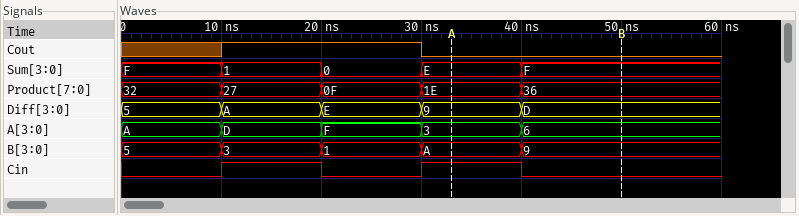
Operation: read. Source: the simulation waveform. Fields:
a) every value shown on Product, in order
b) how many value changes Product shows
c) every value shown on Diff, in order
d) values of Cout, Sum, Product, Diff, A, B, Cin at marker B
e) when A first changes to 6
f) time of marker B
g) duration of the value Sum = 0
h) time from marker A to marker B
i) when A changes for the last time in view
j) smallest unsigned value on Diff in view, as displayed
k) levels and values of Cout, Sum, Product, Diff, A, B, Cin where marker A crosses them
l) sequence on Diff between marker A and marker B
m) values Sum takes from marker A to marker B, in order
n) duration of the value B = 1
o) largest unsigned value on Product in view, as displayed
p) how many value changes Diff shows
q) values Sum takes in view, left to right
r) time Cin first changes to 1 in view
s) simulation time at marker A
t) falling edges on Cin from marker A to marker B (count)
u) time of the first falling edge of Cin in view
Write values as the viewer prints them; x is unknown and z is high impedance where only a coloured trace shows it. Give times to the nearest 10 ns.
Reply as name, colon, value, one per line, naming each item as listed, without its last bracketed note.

every value shown on Product, in order: 32, 27, 0F, 1E, 36
how many value changes Product shows: 4
every value shown on Diff, in order: 5, A, E, 9, D
values of Cout, Sum, Product, Diff, A, B, Cin at marker B: Cout=0, Sum=F, Product=36, Diff=D, A=6, B=9, Cin=0
when A first changes to 6: 40 ns
time of marker B: 50 ns
duration of the value Sum = 0: 10 ns
time from marker A to marker B: 20 ns
when A changes for the last time in view: 40 ns
smallest unsigned value on Diff in view, as displayed: 5
levels and values of Cout, Sum, Product, Diff, A, B, Cin where marker A crosses them: Cout=0, Sum=E, Product=1E, Diff=9, A=3, B=A, Cin=1
sequence on Diff between marker A and marker B: 9, D
values Sum takes from marker A to marker B, in order: E, F
duration of the value B = 1: 10 ns
largest unsigned value on Product in view, as displayed: 36
how many value changes Diff shows: 4
values Sum takes in view, left to right: F, 1, 0, E, F
time Cin first changes to 1 in view: 10 ns
simulation time at marker A: 30 ns
falling edges on Cin from marker A to marker B: 1
time of the first falling edge of Cin in view: 20 ns
